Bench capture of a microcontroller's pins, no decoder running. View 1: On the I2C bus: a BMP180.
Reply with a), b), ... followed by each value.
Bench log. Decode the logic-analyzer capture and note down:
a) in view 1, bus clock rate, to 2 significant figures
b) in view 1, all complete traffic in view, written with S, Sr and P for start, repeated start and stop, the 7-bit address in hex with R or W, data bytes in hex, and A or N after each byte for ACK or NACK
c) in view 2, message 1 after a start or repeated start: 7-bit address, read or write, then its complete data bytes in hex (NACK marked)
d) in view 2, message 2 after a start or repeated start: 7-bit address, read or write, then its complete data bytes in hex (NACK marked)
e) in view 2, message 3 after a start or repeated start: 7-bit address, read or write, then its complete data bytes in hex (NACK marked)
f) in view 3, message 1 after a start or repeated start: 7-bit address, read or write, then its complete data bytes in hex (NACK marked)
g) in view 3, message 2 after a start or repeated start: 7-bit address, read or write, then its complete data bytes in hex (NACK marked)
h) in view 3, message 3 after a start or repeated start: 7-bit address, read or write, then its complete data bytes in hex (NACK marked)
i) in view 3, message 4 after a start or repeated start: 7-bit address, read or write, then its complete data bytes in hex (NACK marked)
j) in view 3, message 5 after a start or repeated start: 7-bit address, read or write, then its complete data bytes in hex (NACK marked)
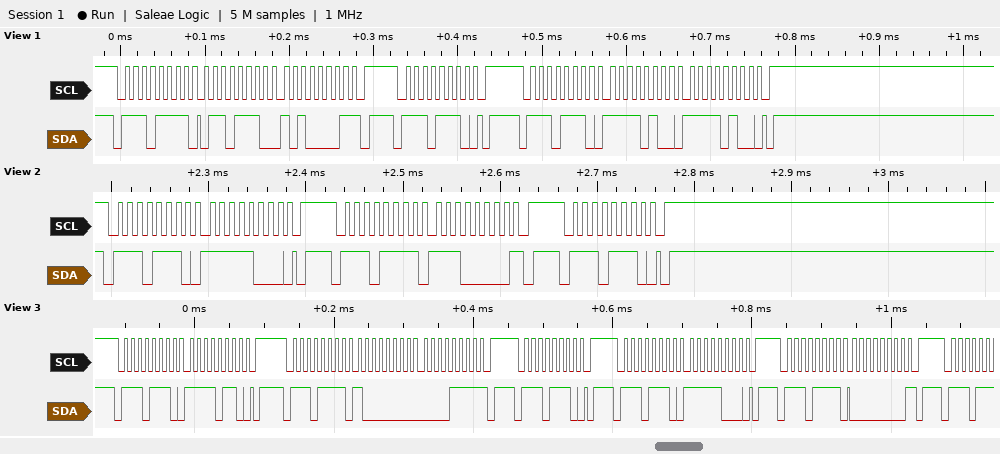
a) 100 kHz
b) S 77R A 6E A A1 N P S 77W A P S 77W A F4 A F4 A P
c) 0x77 write: F8
d) 0x77 read: E0 NACK
e) 0x77 write
f) 0x77 write: F6
g) 0x77 read: 80 0F NACK
h) 0x77 write
i) 0x77 write: F8
j) 0x77 read: 00 NACK
